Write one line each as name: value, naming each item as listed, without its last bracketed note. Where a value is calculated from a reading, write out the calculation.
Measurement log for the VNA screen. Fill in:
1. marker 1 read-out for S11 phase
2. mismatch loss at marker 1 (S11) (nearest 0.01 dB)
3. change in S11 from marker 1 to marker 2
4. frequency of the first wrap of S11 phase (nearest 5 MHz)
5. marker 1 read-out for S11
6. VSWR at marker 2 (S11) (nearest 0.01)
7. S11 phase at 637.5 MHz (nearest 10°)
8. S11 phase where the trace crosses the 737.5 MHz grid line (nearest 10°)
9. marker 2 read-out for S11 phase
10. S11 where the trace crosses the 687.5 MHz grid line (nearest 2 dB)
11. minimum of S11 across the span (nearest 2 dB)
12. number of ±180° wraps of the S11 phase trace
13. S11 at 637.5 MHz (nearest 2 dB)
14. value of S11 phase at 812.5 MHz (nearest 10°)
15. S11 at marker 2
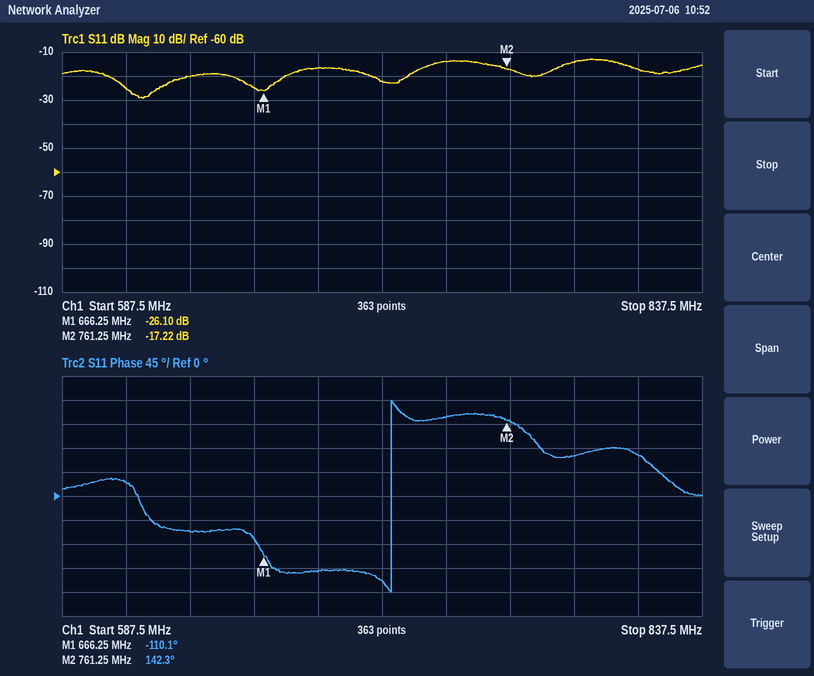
marker 1 read-out for S11 phase: -110.1°
mismatch loss at marker 1 (S11): −10 log10(1 − 10^(-26.1/10)) ≈ 0.01 dB
change in S11 from marker 1 to marker 2: -17.22 − (-26.1) = 8.88 dB
frequency of the first wrap of S11 phase: 715 MHz
marker 1 read-out for S11: -26.10 dB
VSWR at marker 2 (S11): (1 + 0.1377)/(1 − 0.1377) ≈ 1.32
S11 phase at 637.5 MHz: -70°
S11 phase where the trace crosses the 737.5 MHz grid line: 150°
marker 2 read-out for S11 phase: 142.3°
S11 where the trace crosses the 687.5 MHz grid line: -16 dB
minimum of S11 across the span: -30 dB
number of ±180° wraps of the S11 phase trace: 1
S11 at 637.5 MHz: -20 dB
value of S11 phase at 812.5 MHz: 80°
S11 at marker 2: -17.22 dB
